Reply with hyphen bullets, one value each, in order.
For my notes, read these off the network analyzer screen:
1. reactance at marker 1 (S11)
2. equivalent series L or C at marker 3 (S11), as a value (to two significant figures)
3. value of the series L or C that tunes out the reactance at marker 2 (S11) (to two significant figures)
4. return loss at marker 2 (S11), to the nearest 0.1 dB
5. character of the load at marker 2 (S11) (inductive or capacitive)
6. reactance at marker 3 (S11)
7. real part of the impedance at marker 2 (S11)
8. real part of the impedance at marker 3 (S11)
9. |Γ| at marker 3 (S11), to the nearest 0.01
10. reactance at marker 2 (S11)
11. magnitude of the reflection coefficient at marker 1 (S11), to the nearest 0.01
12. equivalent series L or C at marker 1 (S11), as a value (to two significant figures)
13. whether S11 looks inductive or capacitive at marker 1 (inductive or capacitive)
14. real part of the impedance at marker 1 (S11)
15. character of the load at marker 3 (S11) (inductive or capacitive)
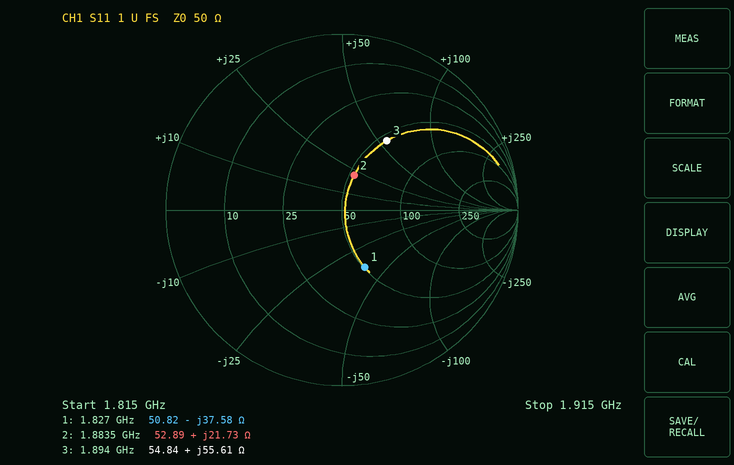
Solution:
- -37.58 Ω
- 4.7 nH
- 3.9 pF
- 13.6 dB
- inductive
- +55.61 Ω
- 52.89 Ω
- 54.84 Ω
- 0.47
- +21.73 Ω
- 0.35
- 2.3 pF
- capacitive
- 50.82 Ω
- inductive
